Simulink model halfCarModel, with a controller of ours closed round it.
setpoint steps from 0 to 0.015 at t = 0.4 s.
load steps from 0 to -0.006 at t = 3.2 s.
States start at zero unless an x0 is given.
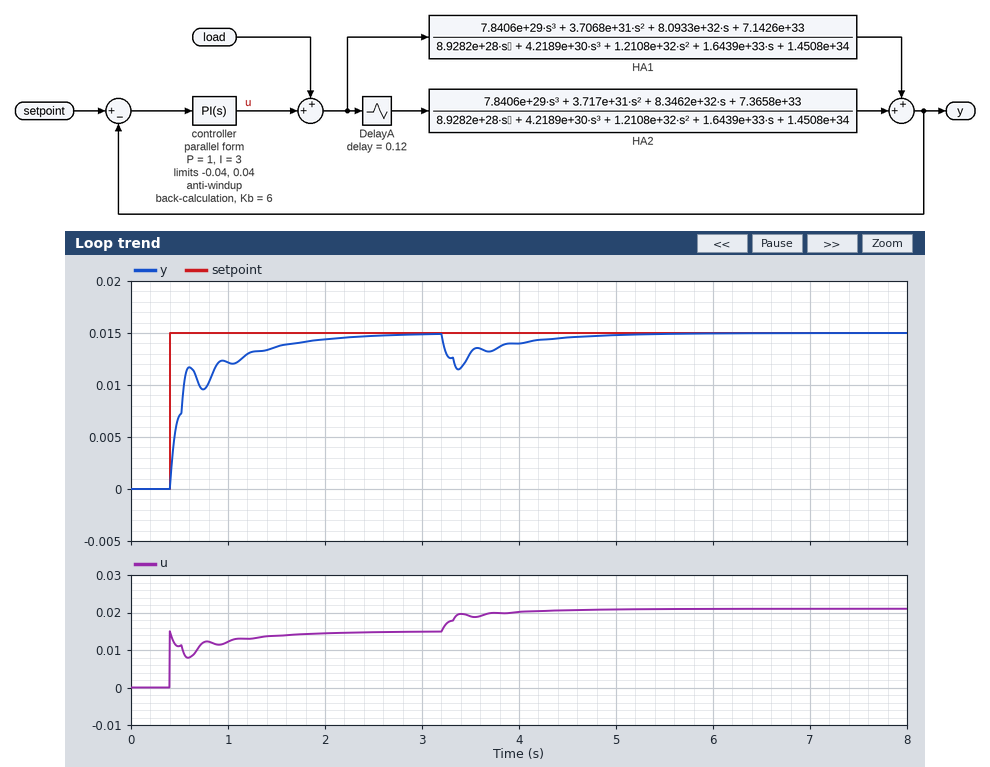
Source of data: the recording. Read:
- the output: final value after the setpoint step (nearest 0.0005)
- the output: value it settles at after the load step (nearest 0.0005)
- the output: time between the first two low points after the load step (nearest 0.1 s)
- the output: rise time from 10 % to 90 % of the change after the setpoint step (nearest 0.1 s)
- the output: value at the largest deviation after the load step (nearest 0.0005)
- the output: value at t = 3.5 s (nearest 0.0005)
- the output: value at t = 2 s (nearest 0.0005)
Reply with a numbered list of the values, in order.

1. 0.0150
2. 0.0150
3. 0.3 s
4. 1.0 s
5. 0.0115
6. 0.0130
7. 0.0145
